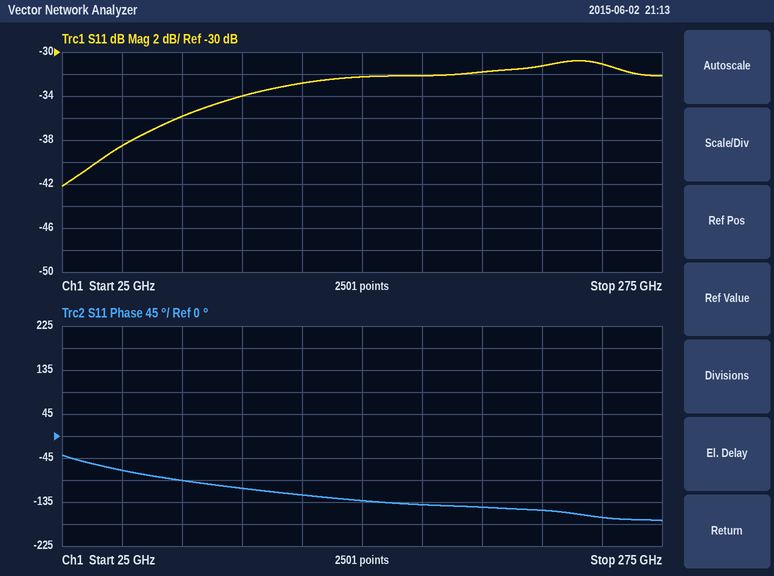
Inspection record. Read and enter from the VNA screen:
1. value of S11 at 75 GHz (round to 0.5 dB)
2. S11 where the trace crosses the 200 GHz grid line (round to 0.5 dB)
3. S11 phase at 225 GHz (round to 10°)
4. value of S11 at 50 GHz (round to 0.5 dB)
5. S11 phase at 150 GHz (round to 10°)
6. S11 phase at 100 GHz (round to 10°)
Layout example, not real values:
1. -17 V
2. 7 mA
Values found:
1. -36.0 dB
2. -32.0 dB
3. -150°
4. -38.5 dB
5. -130°
6. -110°
